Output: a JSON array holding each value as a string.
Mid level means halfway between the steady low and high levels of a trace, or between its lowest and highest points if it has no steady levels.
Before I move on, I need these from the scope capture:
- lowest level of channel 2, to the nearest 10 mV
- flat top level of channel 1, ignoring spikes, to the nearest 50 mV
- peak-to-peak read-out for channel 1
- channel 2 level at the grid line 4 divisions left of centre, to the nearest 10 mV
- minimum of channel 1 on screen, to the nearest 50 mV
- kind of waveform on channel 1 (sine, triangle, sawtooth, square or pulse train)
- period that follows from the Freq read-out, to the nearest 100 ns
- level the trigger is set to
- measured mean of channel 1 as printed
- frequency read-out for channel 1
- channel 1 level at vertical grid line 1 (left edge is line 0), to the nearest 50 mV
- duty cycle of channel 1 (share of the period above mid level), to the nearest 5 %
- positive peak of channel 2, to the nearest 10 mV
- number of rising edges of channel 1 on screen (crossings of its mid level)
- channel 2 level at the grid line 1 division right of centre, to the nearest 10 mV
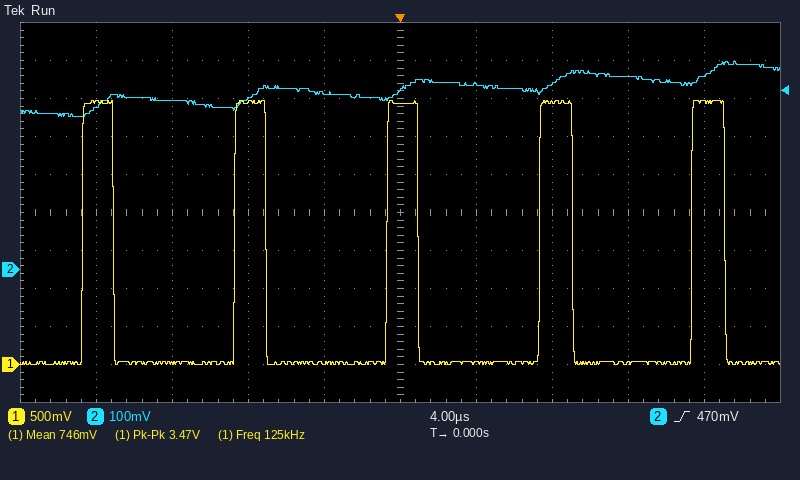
["400 mV", "3.45 V", "3.47 V", "430 mV", "0 mV", "pulse train", "8.0 µs", "470 mV", "746 mV", "125 kHz", "3.45 V", "20 %", "550 mV", "5", "490 mV"]
